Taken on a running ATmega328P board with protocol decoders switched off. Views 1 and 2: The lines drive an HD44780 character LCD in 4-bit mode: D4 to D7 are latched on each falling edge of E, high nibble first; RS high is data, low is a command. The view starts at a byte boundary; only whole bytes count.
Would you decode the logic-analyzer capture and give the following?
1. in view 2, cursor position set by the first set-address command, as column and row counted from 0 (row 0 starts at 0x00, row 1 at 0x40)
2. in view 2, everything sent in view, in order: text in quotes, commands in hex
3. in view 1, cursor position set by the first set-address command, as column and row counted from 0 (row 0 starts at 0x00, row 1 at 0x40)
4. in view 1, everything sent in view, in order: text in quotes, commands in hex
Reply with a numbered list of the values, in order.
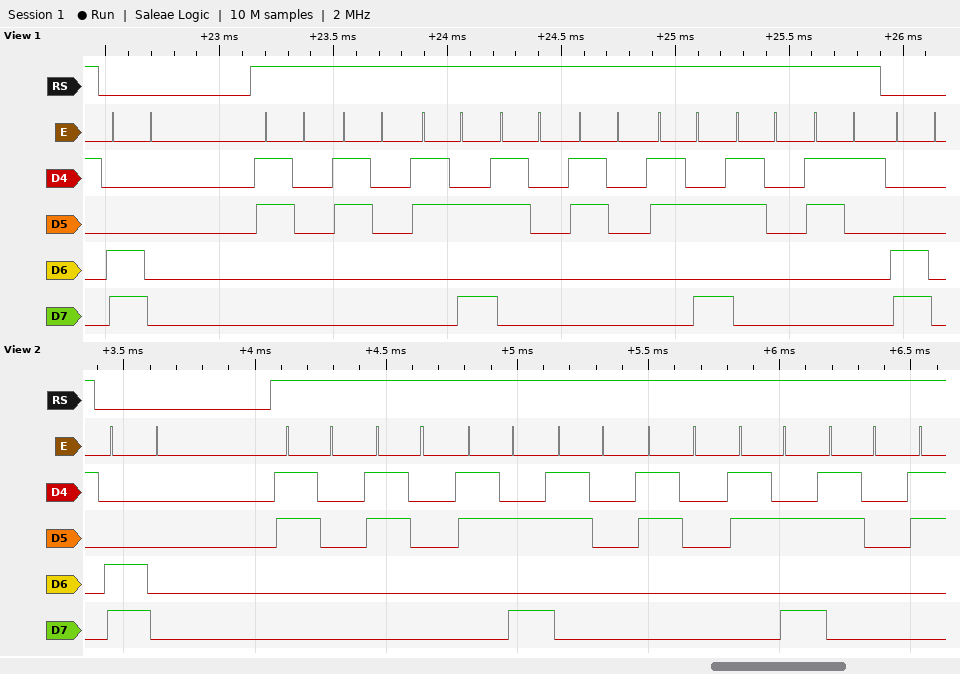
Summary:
1. column 0, row 1
2. 0xC0 "00:00:0"
3. column 0, row 1
4. 0xC0 "00:00:01" 0xC0
